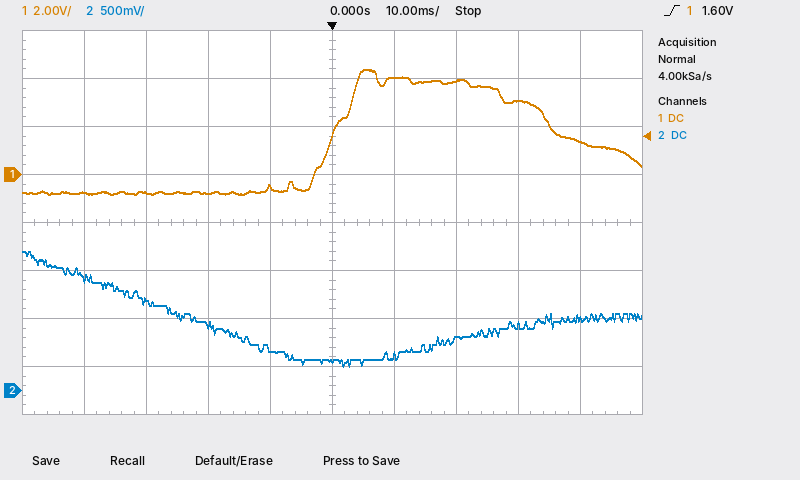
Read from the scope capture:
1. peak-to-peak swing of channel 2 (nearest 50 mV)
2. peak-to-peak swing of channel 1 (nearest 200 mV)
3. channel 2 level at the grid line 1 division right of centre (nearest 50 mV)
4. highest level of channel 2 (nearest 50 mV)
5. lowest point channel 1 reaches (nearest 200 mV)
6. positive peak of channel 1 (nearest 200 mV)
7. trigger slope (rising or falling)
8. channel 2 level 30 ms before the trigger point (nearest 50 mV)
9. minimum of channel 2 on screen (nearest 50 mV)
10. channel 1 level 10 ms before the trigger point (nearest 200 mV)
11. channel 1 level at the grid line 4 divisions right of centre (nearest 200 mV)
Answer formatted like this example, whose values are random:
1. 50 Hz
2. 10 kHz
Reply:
1. 1.20 V
2. 5.2 V
3. 350 mV
4. 1.45 V
5. -800 mV
6. 4.4 V
7. rising
8. 950 mV
9. 250 mV
10. -600 mV
11. 1.4 V
